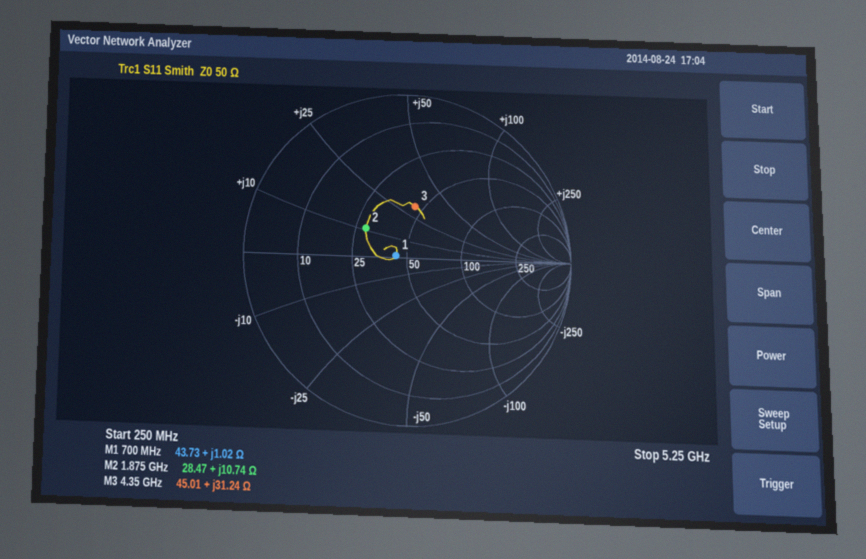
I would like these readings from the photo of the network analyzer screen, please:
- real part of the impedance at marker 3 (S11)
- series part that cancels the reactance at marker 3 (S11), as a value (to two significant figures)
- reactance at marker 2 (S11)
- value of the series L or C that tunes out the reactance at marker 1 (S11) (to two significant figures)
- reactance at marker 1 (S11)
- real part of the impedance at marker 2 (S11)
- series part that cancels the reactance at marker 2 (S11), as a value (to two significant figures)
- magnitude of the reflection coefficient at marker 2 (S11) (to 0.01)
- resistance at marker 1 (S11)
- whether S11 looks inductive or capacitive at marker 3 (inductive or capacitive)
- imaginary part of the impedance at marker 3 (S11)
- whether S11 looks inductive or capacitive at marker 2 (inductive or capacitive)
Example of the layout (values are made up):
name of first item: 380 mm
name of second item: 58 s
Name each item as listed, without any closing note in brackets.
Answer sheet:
real part of the impedance at marker 3: 45.01 Ω
series part that cancels the reactance at marker 3 (S11), as a value: 1.2 pF
reactance at marker 2: +10.74 Ω
value of the series L or C that tunes out the reactance at marker 1 (S11): 220 pF
reactance at marker 1: +1.02 Ω
real part of the impedance at marker 2: 28.47 Ω
series part that cancels the reactance at marker 2 (S11), as a value: 7.9 pF
magnitude of the reflection coefficient at marker 2 (S11): 0.30
resistance at marker 1: 43.73 Ω
whether S11 looks inductive or capacitive at marker 3: inductive
imaginary part of the impedance at marker 3: +31.24 Ω
whether S11 looks inductive or capacitive at marker 2: inductive
